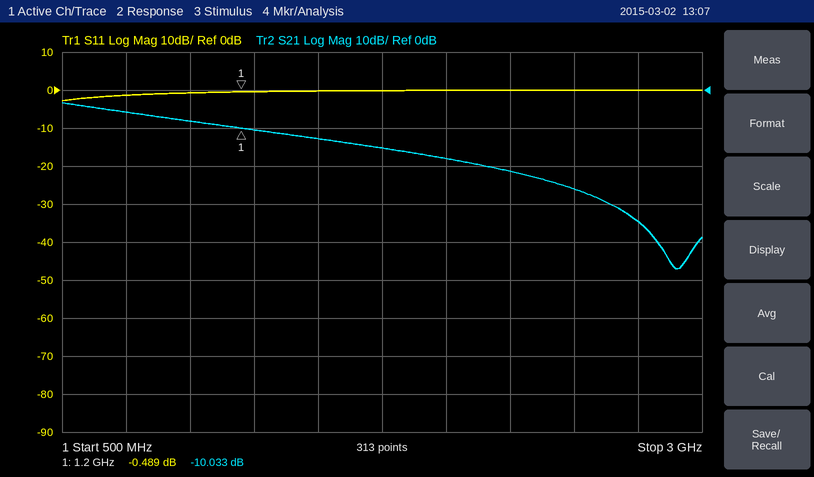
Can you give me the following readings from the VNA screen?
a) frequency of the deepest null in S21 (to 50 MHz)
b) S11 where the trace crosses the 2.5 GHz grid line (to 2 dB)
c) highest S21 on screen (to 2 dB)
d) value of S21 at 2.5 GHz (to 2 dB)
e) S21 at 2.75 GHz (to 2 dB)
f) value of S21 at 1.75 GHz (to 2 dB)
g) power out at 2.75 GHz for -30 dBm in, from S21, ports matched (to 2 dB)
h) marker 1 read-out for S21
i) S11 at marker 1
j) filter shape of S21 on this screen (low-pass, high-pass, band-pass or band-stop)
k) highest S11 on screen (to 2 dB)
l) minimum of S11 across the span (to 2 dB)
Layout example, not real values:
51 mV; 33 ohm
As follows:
2.90 GHz; 0 dB; -4 dB; -26 dB; -34 dB; -16 dB; -64 dBm; -10.033 dB; -0.489 dB; low-pass; 0 dB; -2 dB
